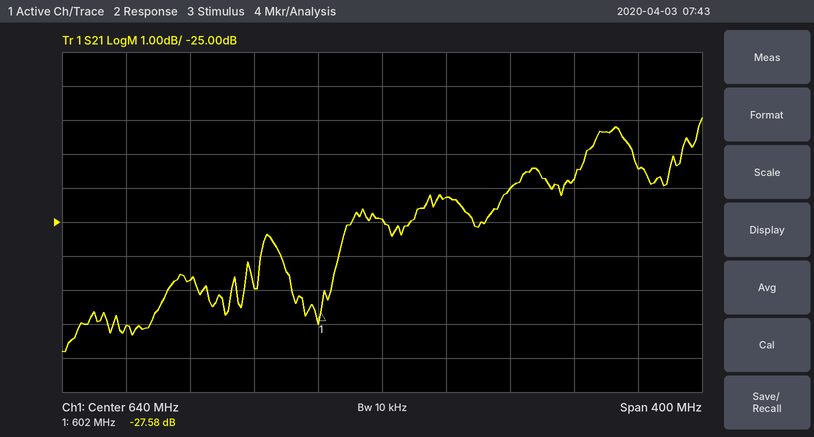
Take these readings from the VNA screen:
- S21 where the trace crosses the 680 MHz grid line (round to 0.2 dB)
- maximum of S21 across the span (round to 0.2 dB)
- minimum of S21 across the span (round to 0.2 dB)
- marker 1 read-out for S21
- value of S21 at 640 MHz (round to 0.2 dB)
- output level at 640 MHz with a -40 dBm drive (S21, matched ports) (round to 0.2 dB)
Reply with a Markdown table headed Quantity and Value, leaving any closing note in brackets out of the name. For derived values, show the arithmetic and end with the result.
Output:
| Quantity | Value |
|---|---|
| S21 where the trace crosses the 680 MHz grid line | -24.2 dB |
| maximum of S21 across the span | -22.0 dB |
| minimum of S21 across the span | -28.8 dB |
| marker 1 read-out for S21 | -27.58 dB |
| value of S21 at 640 MHz | -25.0 dB |
| output level at 640 MHz with a -40 dBm drive (S21, matched ports) | -40 dBm + (-25.0 dB) = -65.0 dBm |
